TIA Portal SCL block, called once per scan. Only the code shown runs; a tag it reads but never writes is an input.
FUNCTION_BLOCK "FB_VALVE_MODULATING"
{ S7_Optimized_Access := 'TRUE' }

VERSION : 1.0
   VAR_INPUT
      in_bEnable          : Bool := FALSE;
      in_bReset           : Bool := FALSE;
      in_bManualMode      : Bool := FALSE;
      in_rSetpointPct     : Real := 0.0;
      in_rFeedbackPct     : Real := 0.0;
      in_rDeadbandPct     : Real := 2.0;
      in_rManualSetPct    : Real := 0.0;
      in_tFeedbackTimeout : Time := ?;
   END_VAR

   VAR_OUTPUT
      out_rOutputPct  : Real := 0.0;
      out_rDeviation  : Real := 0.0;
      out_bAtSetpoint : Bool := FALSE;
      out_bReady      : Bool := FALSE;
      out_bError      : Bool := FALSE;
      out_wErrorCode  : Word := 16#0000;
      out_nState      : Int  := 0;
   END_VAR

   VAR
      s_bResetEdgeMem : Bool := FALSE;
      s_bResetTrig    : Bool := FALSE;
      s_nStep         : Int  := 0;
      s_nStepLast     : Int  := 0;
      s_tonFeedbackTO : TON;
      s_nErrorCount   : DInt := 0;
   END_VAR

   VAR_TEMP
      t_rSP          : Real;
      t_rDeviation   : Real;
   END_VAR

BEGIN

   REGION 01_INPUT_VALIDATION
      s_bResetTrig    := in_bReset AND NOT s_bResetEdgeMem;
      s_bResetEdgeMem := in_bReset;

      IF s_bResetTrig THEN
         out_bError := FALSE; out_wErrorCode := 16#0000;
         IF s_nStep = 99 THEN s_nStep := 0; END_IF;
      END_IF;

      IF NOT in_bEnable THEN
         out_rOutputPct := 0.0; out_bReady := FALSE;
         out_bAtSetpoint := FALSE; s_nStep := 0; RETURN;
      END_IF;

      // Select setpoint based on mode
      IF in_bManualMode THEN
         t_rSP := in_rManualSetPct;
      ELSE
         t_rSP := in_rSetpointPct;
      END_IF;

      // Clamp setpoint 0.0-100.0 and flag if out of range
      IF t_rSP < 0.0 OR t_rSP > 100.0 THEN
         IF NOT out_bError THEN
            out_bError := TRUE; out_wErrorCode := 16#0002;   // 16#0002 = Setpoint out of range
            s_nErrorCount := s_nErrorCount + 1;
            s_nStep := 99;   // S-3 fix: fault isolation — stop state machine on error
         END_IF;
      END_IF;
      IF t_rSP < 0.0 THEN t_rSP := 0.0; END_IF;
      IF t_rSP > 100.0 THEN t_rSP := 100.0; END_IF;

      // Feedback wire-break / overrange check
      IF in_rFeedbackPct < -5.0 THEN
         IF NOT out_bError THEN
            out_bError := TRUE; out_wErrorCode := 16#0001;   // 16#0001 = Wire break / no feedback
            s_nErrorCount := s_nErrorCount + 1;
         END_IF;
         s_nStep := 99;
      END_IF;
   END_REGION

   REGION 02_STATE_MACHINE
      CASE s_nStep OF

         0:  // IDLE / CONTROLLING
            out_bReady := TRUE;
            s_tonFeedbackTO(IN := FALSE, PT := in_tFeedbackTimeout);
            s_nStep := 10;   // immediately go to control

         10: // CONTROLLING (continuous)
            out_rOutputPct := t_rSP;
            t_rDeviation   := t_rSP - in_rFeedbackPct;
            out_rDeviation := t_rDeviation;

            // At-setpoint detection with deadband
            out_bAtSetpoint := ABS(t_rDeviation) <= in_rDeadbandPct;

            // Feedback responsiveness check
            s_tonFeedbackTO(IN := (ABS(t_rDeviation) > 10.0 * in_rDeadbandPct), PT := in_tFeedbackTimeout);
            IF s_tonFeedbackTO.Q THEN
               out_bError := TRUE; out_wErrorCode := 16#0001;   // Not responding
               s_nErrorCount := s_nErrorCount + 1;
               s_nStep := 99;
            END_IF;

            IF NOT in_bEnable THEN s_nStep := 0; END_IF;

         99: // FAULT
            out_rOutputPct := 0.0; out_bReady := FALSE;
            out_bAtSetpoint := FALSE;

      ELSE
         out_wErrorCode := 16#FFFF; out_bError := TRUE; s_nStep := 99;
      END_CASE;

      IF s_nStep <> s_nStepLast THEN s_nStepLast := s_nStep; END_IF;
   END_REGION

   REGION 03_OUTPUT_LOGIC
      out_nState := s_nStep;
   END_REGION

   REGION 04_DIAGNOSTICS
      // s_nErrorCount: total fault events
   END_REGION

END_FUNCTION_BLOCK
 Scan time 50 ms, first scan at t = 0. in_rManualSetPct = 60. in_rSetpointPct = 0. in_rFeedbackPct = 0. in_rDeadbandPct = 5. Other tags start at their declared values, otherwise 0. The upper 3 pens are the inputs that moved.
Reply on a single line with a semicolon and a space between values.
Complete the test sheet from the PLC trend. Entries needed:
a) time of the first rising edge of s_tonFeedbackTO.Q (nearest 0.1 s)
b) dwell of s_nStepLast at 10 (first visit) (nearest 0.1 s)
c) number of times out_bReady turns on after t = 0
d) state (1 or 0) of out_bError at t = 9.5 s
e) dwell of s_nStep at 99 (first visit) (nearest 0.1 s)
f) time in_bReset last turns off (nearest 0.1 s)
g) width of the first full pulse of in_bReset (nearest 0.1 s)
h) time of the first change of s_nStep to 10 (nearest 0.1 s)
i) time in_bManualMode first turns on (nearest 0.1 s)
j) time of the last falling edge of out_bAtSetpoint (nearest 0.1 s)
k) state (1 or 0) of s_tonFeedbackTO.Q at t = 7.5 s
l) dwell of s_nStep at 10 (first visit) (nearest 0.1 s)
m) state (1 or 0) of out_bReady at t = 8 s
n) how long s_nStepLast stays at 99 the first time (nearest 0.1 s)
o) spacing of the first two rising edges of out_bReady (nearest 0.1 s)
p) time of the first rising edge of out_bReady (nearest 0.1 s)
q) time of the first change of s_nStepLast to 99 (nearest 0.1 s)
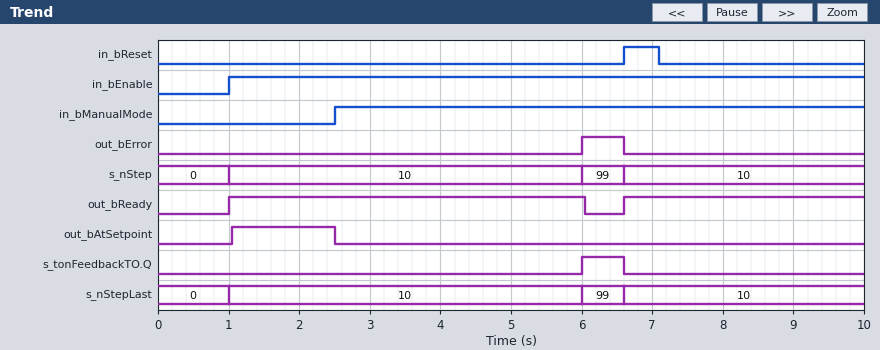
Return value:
6.0 s; 5.0 s; 2; 0; 0.6 s; 7.1 s; 0.5 s; 1.0 s; 2.5 s; 2.5 s; 0; 5.0 s; 1; 0.6 s; 5.6 s; 1.0 s; 6.0 s
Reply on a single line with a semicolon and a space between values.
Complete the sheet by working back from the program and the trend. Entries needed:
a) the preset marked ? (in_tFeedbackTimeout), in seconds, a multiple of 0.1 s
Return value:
3.5 s
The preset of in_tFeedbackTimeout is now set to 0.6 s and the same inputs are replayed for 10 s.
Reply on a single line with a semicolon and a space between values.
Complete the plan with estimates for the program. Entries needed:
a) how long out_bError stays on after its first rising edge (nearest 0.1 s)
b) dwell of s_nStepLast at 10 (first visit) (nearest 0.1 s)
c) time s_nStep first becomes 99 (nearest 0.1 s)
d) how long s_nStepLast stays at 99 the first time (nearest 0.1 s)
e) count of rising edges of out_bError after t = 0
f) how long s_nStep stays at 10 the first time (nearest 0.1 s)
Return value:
3.5 s; 2.1 s; 3.1 s; 3.5 s; 2; 2.1 s
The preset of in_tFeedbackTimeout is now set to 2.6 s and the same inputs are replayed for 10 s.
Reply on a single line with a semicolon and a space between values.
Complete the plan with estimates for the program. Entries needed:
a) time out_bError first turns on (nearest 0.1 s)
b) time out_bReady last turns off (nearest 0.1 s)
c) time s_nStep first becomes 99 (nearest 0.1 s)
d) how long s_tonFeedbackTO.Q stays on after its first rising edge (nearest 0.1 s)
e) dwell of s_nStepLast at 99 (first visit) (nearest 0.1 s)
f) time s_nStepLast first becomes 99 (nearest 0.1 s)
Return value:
5.1 s; 9.3 s; 5.1 s; 1.5 s; 1.5 s; 5.1 s
